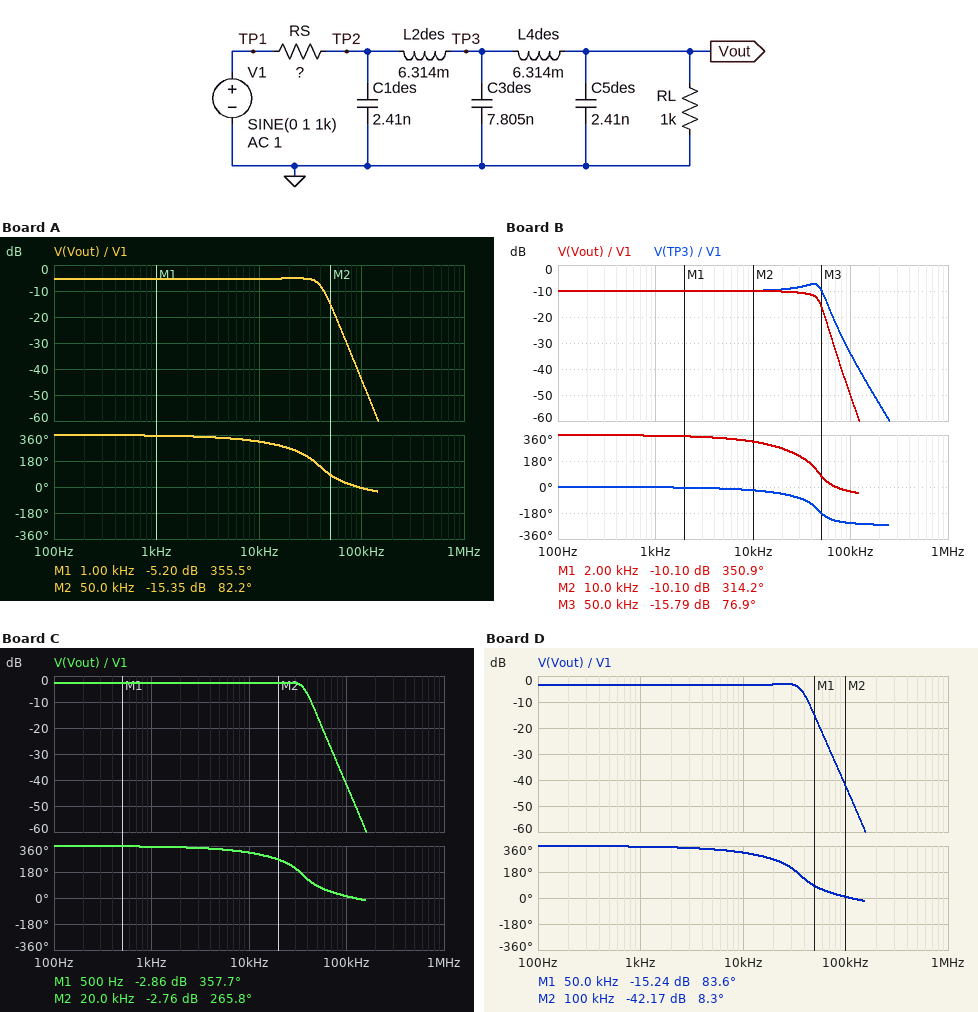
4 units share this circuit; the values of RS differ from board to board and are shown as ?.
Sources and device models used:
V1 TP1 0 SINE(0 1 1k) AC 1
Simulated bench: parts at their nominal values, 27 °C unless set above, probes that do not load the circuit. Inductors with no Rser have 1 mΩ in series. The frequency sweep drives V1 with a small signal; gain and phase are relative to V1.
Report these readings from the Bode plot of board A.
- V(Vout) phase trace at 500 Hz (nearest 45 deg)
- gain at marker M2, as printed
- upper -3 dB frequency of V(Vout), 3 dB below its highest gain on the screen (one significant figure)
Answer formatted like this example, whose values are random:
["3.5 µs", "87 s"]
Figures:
["360 deg", "-15.35 dB", "40 kHz"]
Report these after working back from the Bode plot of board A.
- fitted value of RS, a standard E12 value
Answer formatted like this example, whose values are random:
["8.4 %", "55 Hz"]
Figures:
["820 Ω"]
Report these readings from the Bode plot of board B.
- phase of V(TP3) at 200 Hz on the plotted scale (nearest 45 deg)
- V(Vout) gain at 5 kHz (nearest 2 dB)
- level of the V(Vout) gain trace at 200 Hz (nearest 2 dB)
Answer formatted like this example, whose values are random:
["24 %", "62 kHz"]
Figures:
["0 deg", "-10 dB", "-10 dB"]
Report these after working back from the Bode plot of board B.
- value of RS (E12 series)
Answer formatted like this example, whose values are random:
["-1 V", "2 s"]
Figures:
["2.2 kΩ"]
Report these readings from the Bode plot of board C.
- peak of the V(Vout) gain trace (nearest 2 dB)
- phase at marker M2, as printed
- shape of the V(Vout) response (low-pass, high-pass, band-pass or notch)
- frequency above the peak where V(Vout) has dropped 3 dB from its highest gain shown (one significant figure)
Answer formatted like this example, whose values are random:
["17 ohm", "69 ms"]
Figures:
["-2 dB", "265.8 deg", "low-pass", "40 kHz"]
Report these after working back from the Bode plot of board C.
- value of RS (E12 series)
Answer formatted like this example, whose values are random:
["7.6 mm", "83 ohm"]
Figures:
["390 Ω"]
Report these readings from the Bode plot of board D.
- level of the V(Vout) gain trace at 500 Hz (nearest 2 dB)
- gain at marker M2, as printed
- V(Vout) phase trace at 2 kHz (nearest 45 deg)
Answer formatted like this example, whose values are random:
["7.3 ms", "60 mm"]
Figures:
["-4 dB", "-42.17 dB", "360 deg"]
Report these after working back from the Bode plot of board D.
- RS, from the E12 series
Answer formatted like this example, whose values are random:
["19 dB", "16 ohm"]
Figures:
["470 Ω"]
